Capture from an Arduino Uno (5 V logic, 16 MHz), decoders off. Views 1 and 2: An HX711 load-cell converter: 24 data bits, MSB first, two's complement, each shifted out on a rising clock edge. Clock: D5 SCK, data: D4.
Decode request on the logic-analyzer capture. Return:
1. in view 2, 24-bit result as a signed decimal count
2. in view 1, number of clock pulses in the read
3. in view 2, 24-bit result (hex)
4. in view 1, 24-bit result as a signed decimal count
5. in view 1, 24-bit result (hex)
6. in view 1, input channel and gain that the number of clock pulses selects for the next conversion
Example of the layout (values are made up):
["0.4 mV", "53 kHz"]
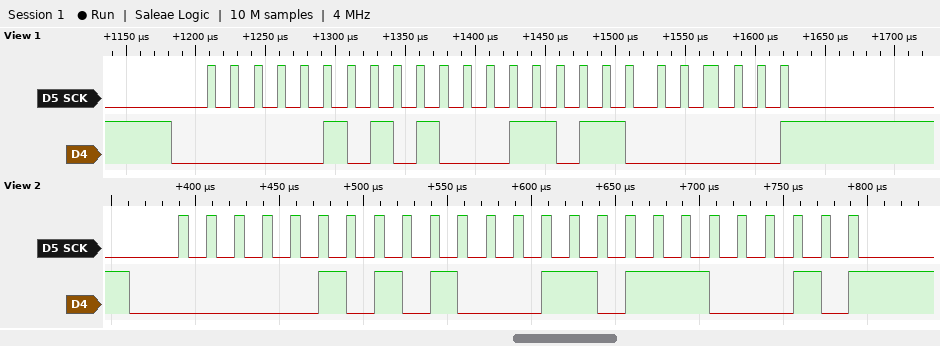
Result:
["345826", "25", "0x0546E2", "345792", "0x0546C0", "channel A, gain 128"]
